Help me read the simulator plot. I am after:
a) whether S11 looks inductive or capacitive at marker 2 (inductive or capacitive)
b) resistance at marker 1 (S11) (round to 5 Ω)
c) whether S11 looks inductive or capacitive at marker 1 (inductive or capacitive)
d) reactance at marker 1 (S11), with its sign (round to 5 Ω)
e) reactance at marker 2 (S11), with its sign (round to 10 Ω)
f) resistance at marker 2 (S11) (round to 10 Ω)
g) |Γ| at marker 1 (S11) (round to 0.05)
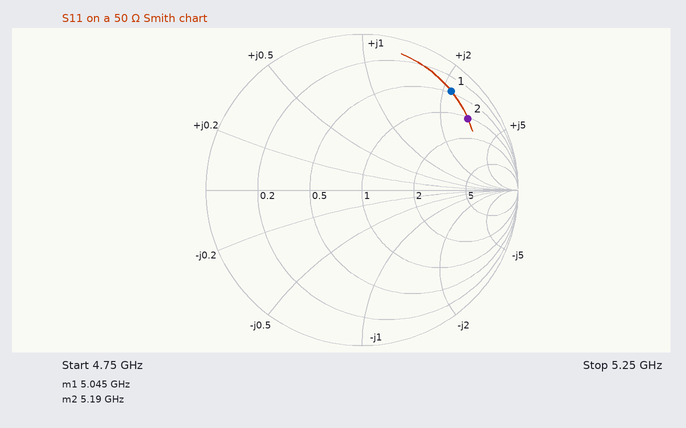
inductive
25 Ω
inductive
+110 Ω
+150 Ω
50 Ω
0.85
